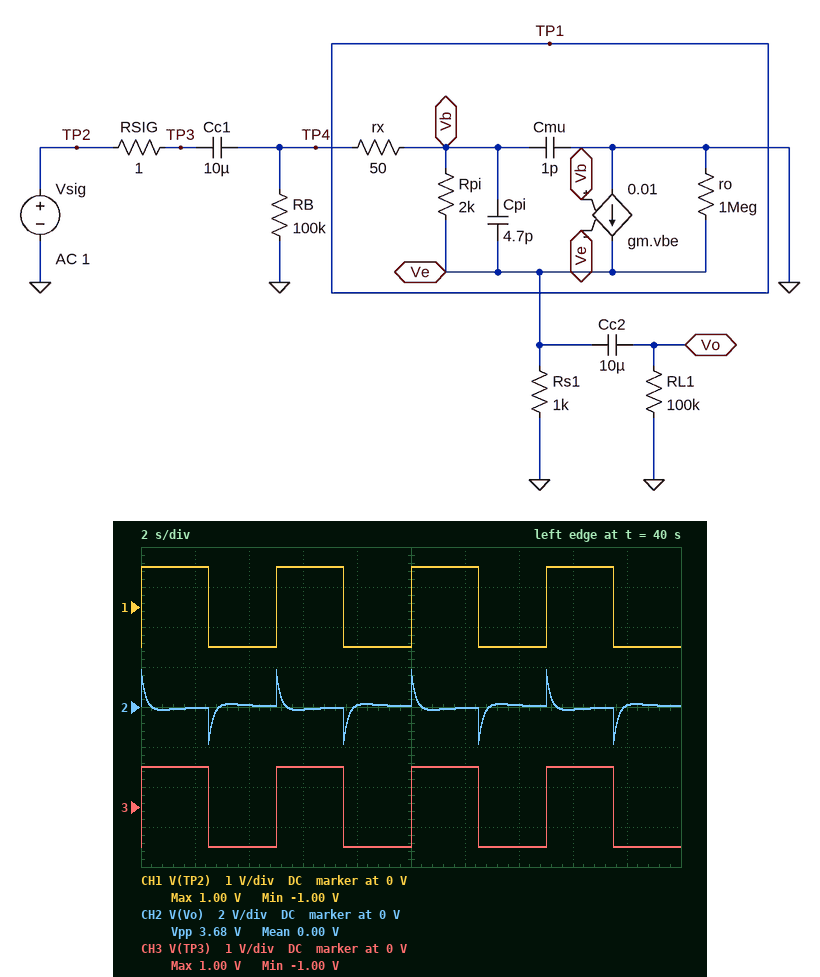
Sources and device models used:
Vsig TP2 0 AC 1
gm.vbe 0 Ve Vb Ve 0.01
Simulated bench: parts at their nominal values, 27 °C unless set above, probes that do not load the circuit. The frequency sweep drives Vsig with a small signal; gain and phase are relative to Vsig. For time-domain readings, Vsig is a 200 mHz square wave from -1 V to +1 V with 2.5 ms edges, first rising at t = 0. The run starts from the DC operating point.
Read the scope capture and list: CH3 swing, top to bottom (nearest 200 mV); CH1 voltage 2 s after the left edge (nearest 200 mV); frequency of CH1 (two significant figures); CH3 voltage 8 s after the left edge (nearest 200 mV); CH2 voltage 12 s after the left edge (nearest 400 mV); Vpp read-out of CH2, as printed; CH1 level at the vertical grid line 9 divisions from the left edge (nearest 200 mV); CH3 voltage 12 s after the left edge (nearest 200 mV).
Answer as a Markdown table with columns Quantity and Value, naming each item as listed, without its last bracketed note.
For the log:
| Quantity | Value |
|---|---|
| CH3 swing, top to bottom | 2.0 V |
| CH1 voltage 2 s after the left edge | 1.0 V |
| frequency of CH1 | 200 mHz |
| CH3 voltage 8 s after the left edge | -1.0 V |
| CH2 voltage 12 s after the left edge | 0 V |
| Vpp read-out of CH2, as printed | 3.68 V |
| CH1 level at the vertical grid line 9 divisions from the left edge | -1.0 V |
| CH3 voltage 12 s after the left edge | 1.0 V |
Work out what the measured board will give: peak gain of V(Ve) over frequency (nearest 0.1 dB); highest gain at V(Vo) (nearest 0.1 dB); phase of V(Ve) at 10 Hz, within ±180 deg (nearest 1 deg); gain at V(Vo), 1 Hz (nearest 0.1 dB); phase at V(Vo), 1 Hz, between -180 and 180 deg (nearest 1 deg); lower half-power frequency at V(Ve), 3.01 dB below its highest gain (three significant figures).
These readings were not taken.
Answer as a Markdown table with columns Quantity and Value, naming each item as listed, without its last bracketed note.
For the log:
| Quantity | Value |
|---|---|
| peak gain of V(Ve) over frequency | -0.8 dB |
| highest gain at V(Vo) | -0.8 dB |
| phase of V(Ve) at 10 Hz, within ±180 deg | 5 deg |
| gain at V(Vo), 1 Hz | -3.3 dB |
| phase at V(Vo), 1 Hz, between -180 and 180 deg | 50 deg |
| lower half-power frequency at V(Ve), 3.01 dB below its highest gain | 857 mHz |
